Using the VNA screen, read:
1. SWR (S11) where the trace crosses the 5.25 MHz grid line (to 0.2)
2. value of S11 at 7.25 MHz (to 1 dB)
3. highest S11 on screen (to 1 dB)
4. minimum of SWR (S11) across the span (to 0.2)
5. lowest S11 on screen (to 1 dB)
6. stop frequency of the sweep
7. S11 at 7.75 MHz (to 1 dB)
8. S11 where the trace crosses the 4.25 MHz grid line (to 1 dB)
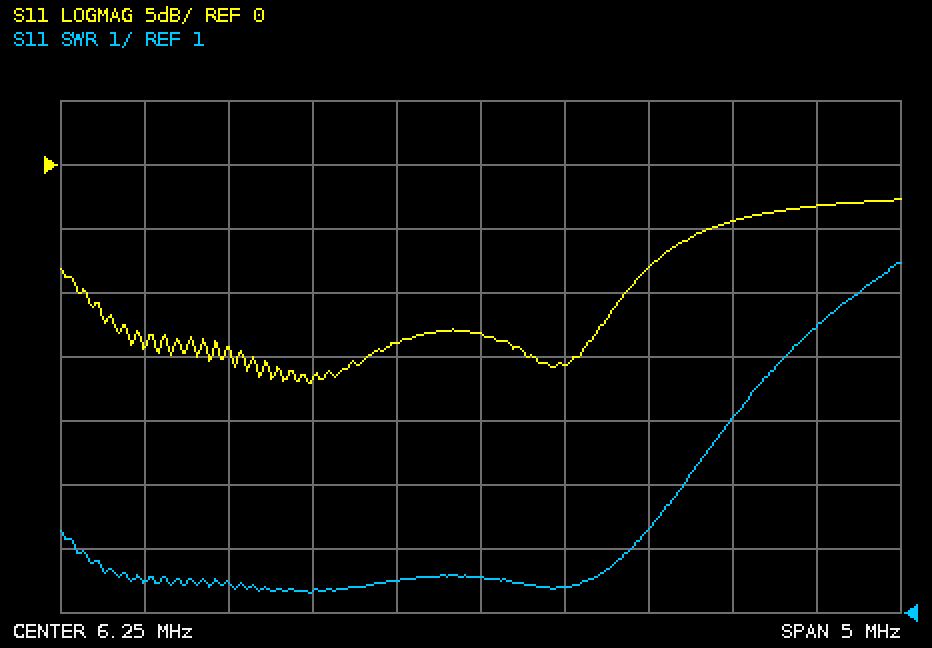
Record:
1.4
-8 dB
-3 dB
1.4
-17 dB
8.75 MHz
-4 dB
-14 dB
